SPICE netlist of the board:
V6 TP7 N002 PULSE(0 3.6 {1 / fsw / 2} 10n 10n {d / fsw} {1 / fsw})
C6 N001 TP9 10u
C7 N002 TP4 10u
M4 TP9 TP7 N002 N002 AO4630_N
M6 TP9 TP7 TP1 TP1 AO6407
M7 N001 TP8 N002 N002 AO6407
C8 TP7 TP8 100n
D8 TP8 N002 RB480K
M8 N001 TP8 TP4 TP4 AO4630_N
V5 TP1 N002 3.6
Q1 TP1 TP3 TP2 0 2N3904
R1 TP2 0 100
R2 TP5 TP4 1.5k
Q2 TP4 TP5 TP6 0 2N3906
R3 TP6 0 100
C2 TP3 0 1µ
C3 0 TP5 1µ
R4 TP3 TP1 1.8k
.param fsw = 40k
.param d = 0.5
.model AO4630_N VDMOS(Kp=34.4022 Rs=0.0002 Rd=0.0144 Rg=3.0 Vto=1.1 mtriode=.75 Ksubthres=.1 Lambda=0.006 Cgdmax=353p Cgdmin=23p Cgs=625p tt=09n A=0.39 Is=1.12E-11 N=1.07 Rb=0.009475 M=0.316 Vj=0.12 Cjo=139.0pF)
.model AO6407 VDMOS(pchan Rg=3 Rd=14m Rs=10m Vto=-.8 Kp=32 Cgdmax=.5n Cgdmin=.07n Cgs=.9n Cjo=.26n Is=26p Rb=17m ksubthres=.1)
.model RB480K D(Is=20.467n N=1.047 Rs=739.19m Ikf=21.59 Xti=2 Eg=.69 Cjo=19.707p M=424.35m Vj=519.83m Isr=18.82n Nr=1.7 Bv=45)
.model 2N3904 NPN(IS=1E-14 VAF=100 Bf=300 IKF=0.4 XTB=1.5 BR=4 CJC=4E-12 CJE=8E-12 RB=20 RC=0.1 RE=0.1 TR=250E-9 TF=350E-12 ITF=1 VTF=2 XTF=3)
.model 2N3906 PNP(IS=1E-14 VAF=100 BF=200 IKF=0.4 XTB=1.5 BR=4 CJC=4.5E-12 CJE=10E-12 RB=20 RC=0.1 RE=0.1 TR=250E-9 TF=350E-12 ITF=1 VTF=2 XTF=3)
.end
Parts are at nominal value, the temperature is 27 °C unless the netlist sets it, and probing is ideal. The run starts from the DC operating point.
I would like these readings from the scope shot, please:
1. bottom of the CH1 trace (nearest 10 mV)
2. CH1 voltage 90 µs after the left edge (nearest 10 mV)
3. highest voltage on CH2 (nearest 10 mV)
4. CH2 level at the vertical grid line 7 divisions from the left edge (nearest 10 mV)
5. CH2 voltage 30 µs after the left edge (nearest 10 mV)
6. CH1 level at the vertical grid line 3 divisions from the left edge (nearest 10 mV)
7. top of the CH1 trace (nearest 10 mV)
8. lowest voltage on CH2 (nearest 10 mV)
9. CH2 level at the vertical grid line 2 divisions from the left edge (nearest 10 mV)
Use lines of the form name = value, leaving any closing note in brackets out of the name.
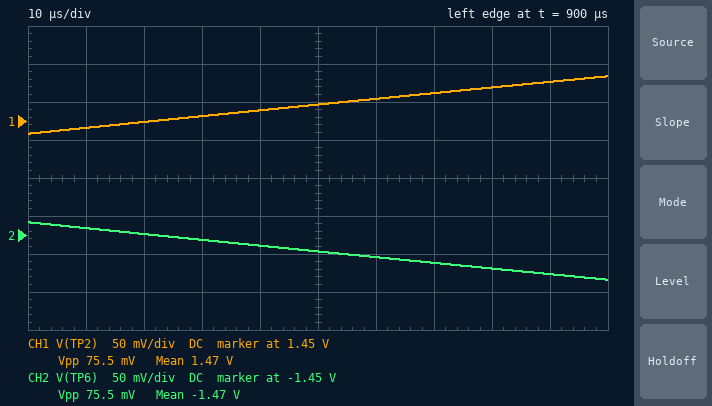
bottom of the CH1 trace = 1.43 V
CH1 voltage 90 µs after the left edge = 1.50 V
highest voltage on CH2 = -1.43 V
CH2 level at the vertical grid line 7 divisions from the left edge = -1.49 V
CH2 voltage 30 µs after the left edge = -1.46 V
CH1 level at the vertical grid line 3 divisions from the left edge = 1.46 V
top of the CH1 trace = 1.51 V
lowest voltage on CH2 = -1.51 V
CH2 level at the vertical grid line 2 divisions from the left edge = -1.45 V
